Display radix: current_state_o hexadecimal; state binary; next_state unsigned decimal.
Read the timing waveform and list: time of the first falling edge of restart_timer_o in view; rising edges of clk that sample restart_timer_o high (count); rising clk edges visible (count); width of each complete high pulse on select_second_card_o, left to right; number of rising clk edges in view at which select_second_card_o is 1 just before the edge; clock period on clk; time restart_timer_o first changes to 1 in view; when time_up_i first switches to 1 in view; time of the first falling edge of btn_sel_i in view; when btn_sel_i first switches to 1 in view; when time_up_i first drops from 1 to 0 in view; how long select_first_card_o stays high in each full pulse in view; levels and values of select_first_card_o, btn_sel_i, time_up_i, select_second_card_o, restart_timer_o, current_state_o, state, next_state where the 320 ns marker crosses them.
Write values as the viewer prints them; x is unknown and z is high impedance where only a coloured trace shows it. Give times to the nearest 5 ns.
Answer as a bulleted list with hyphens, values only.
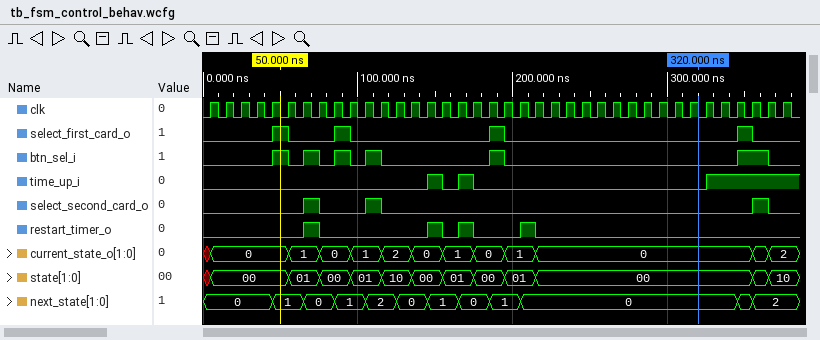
- 75 ns
- 4
- 38
- 10 ns, 10 ns, 10 ns
- 3
- 10 ns
- 65 ns
- 145 ns
- 55 ns
- 45 ns
- 155 ns
- 10 ns, 10 ns, 10 ns, 10 ns
- select_first_card_o=0, btn_sel_i=0, time_up_i=0, select_second_card_o=0, restart_timer_o=0, current_state_o=0, state=00, next_state=0
